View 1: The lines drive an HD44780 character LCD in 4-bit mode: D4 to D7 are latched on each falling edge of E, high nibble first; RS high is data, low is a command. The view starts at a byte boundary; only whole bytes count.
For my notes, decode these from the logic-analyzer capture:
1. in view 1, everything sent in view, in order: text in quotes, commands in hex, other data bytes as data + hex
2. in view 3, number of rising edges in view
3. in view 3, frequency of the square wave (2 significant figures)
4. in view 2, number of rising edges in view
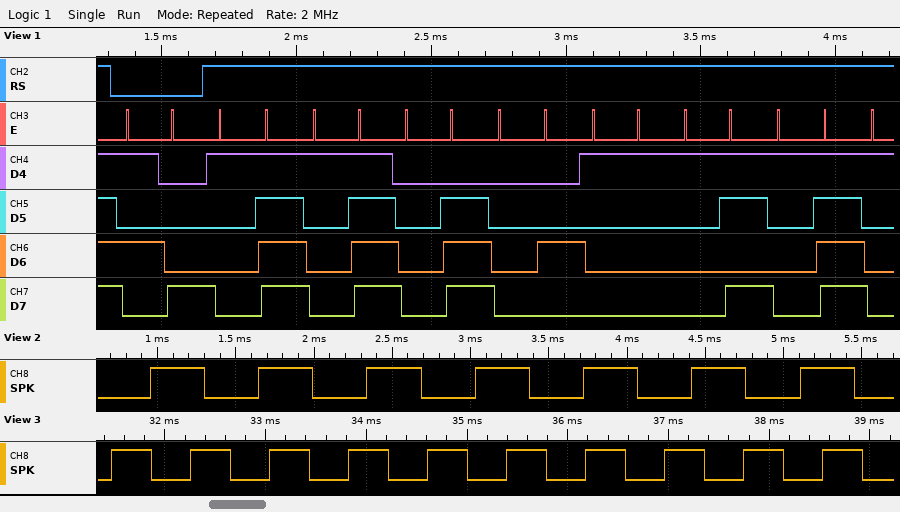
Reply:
0x58 data 1F 1F 0E 04 11 1B 1F
10
1.3 kHz
7
